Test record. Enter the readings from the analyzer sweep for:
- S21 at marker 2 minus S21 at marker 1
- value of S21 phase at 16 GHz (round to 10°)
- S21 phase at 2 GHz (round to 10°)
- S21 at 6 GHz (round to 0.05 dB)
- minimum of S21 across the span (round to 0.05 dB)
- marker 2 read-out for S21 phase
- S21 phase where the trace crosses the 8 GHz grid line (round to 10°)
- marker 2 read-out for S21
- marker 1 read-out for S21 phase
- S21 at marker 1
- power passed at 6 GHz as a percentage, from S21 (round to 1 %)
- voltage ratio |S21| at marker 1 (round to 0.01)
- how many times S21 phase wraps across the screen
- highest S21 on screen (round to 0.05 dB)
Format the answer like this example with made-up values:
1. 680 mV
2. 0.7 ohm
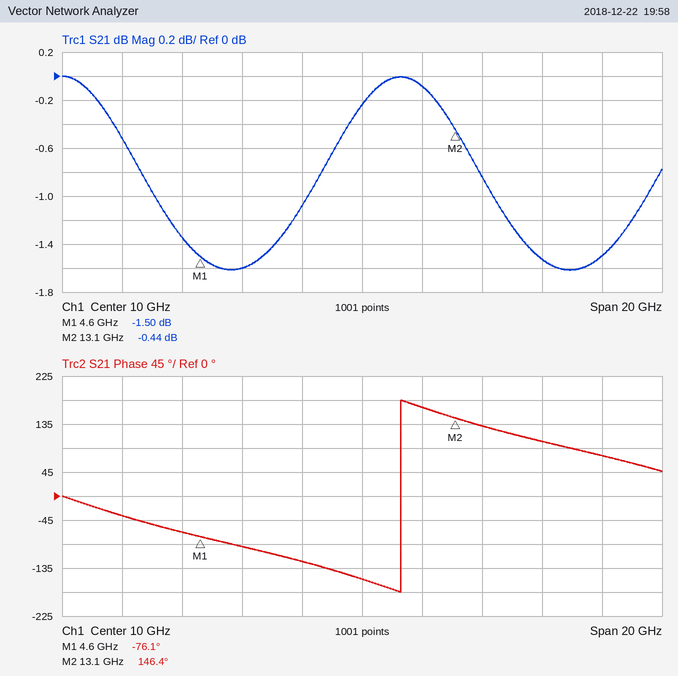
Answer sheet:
1. 1.06 dB
2. 100°
3. -40°
4. -1.60 dB
5. -1.60 dB
6. 146.4°
7. -120°
8. -0.44 dB
9. -76.1°
10. -1.50 dB
11. 69 %
12. 0.84
13. 1
14. 0.00 dB
